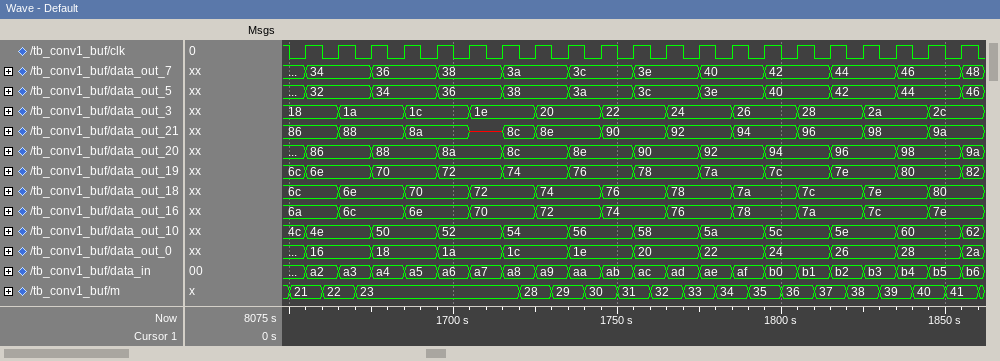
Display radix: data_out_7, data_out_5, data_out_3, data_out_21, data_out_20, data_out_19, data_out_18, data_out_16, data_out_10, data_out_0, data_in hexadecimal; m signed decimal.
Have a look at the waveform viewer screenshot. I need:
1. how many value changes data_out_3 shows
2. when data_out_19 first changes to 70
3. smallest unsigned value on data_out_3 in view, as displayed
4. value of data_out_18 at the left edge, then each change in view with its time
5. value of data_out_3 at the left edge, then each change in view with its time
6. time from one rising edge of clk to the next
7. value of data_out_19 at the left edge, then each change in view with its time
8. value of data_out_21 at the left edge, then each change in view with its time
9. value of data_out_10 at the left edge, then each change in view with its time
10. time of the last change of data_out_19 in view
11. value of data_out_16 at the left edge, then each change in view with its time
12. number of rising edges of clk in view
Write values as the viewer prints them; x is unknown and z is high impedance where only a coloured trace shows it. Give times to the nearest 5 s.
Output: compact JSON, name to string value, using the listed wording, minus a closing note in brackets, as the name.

{"how many value changes data_out_3 shows": "10", "when data_out_19 first changes to 70": "1675 s", "smallest unsigned value on data_out_3 in view, as displayed": "18", "value of data_out_18 at the left edge, then each change in view with its time": "6c, 6e at 1665 s, 70 at 1685 s, 72 at 1705 s, 74 at 1725 s, 76 at 1745 s, 78 at 1765 s, 7a at 1785 s, 7c at 1805 s, 7e at 1825 s, 80 at 1845 s", "value of data_out_3 at the left edge, then each change in view with its time": "18, 1a at 1665 s, 1c at 1685 s, 1e at 1705 s, 20 at 1725 s, 22 at 1745 s, 24 at 1765 s, 26 at 1785 s, 28 at 1805 s, 2a at 1825 s, 2c at 1845 s", "time from one rising edge of clk to the next": "10 s", "value of data_out_19 at the left edge, then each change in view with its time": "6c, 6e at 1655 s, 70 at 1675 s, 72 at 1695 s, 74 at 1715 s, 76 at 1735 s, 78 at 1755 s, 7a at 1775 s, 7c at 1795 s, 7e at 1815 s, 80 at 1835 s, 82 at 1855 s", "value of data_out_21 at the left edge, then each change in view with its time": "86, 88 at 1665 s, 8a at 1685 s, x at 1705 s, 8c at 1715 s, 8e at 1725 s, 90 at 1745 s, 92 at 1765 s, 94 at 1785 s, 96 at 1805 s, 98 at 1825 s, 9a at 1845 s", "value of data_out_10 at the left edge, then each change in view with its time": "4c, 4e at 1655 s, 50 at 1675 s, 52 at 1695 s, 54 at 1715 s, 56 at 1735 s, 58 at 1755 s, 5a at 1775 s, 5c at 1795 s, 5e at 1815 s, 60 at 1835 s, 62 at 1855 s", "time of the last change of data_out_19 in view": "1855 s", "value of data_out_16 at the left edge, then each change in view with its time": "6a, 6c at 1665 s, 6e at 1685 s, 70 at 1705 s, 72 at 1725 s, 74 at 1745 s, 76 at 1765 s, 78 at 1785 s, 7a at 1805 s, 7c at 1825 s, 7e at 1845 s", "number of rising edges of clk in view": "21"}
